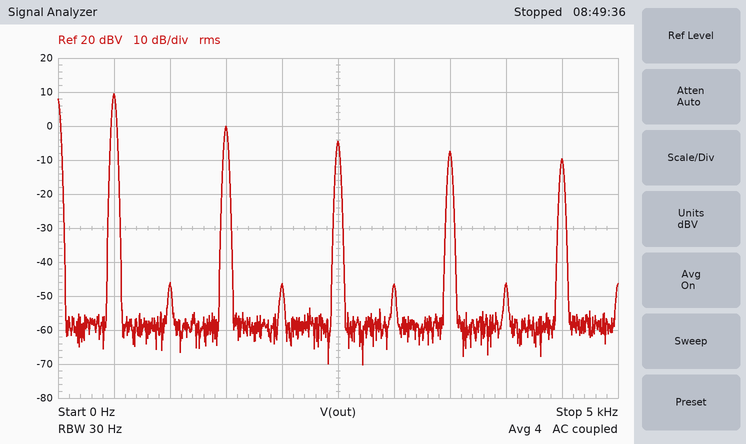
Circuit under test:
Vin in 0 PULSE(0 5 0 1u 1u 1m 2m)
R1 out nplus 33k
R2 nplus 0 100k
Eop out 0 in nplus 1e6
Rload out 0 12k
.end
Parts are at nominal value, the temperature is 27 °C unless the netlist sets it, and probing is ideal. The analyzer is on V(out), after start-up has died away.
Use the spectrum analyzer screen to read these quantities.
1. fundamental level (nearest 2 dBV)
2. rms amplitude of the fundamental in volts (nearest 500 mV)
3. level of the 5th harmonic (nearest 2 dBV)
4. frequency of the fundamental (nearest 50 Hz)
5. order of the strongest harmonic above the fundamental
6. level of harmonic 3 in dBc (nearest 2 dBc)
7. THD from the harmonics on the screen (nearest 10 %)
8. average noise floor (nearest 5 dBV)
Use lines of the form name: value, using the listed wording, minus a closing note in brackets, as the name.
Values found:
fundamental level: 10 dBV
rms amplitude of the fundamental in volts: 3.0 V
level of the 5th harmonic: -4 dBV
frequency of the fundamental: 500 Hz
order of the strongest harmonic above the fundamental: 3
level of harmonic 3 in dBc: -10 dBc
THD from the harmonics on the screen: 40 %
average noise floor: -60 dBV
